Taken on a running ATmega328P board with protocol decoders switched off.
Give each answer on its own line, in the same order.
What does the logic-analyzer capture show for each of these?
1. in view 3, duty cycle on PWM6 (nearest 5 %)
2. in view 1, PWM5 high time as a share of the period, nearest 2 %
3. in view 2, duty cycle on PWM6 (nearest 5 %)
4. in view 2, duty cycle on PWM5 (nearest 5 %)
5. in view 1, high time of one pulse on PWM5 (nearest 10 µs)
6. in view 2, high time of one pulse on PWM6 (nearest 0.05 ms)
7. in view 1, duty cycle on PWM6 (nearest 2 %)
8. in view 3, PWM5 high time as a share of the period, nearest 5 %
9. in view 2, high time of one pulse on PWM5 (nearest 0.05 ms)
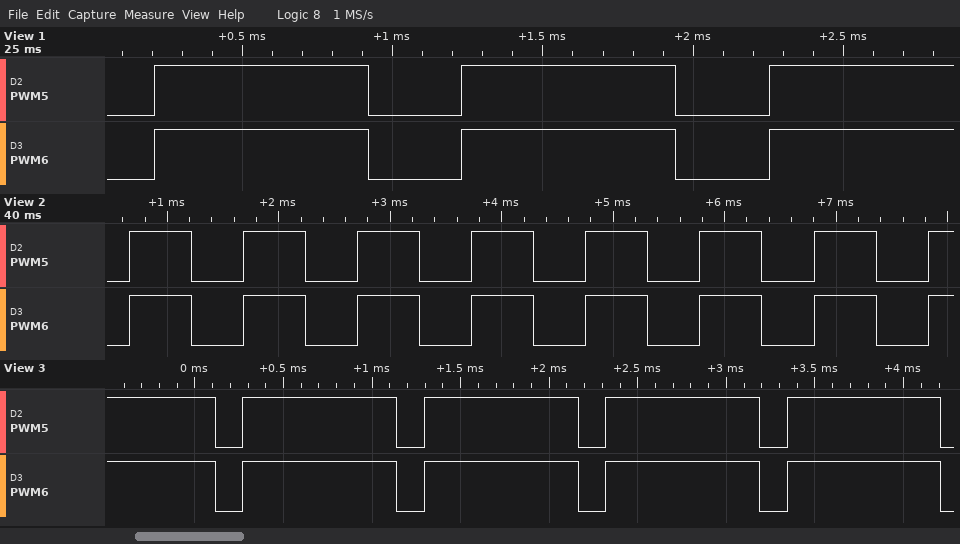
85 %
70 %
55 %
55 %
710 µs
0.55 ms
70 %
85 %
0.55 ms
